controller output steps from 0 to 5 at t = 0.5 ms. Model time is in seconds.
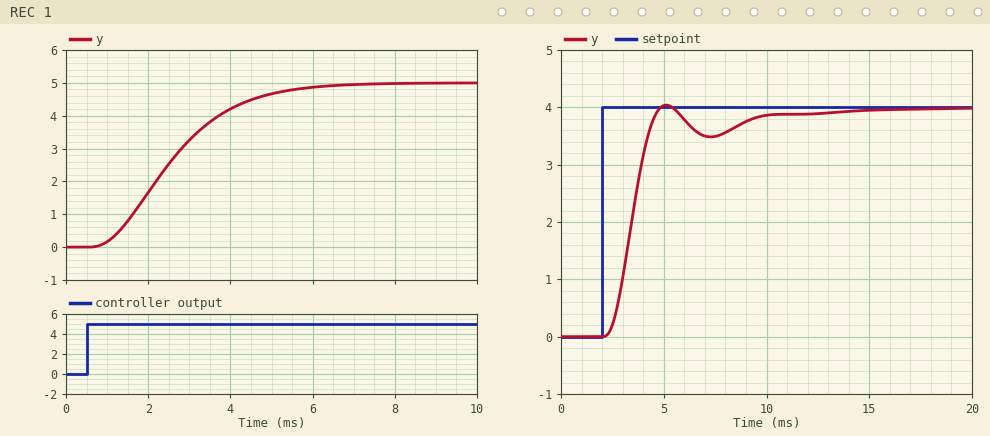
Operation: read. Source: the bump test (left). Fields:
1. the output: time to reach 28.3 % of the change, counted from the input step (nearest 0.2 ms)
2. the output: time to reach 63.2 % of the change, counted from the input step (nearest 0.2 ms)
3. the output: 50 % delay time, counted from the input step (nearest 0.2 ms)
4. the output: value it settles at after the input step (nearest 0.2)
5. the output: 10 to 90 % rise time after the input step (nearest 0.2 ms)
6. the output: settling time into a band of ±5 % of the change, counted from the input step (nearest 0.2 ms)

1.4 ms
2.4 ms
2.0 ms
5.0
3.2 ms
4.8 ms
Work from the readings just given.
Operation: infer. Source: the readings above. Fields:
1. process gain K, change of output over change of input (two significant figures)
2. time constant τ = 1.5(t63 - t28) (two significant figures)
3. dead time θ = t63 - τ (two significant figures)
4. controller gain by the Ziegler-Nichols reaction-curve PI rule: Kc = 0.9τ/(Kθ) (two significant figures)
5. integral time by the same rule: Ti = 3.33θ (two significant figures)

1.0
1.5 ms
0.90 ms
1.5
3.0 ms
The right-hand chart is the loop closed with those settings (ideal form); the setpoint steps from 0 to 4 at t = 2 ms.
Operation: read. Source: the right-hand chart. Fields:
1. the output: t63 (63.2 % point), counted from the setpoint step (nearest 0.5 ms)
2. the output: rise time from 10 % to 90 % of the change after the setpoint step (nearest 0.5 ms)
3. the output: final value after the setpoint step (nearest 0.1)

1.5 ms
1.5 ms
4.0
